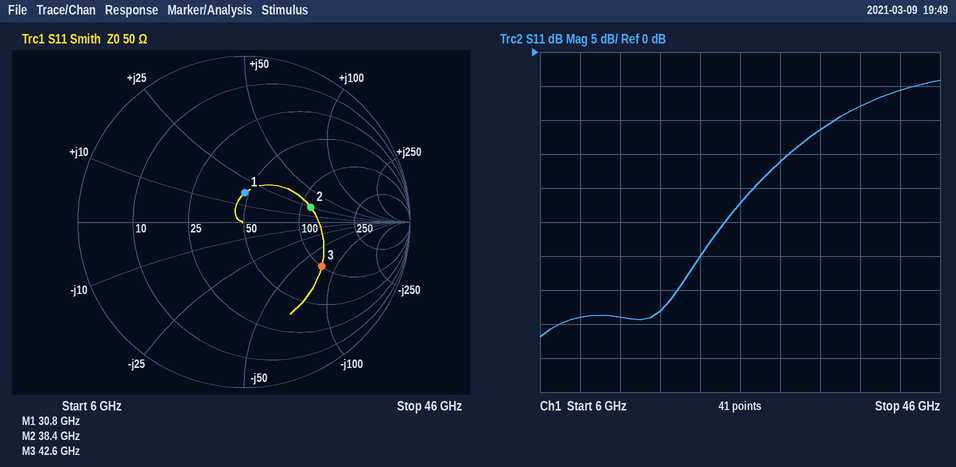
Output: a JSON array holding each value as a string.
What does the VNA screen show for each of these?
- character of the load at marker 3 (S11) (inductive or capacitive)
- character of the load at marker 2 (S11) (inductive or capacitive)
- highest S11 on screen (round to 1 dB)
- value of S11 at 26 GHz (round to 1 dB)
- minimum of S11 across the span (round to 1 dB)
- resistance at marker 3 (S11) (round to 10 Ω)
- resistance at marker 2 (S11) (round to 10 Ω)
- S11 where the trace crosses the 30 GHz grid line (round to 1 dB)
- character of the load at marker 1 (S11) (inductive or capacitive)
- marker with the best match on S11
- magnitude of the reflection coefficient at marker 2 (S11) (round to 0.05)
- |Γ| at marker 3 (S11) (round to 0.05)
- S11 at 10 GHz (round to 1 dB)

["capacitive", "inductive", "-4 dB", "-22 dB", "-42 dB", "100 Ω", "110 Ω", "-16 dB", "inductive", "marker 1", "0.40", "0.55", "-39 dB"]
